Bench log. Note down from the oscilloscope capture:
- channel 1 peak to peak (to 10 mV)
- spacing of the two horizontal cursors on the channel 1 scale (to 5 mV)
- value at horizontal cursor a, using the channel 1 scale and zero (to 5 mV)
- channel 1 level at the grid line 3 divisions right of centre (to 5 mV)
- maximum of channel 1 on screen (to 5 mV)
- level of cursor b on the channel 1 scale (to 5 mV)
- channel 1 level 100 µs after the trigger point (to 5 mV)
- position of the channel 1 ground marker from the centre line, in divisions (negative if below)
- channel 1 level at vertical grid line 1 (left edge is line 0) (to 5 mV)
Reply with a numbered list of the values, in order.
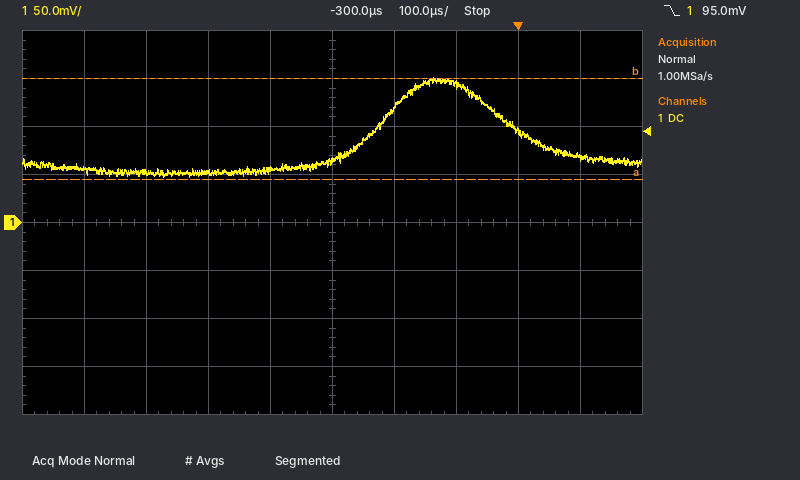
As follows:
1. 100 mV
2. 105 mV
3. 45 mV
4. 95 mV
5. 150 mV
6. 150 mV
7. 70 mV
8. 0.0 div
9. 55 mV
